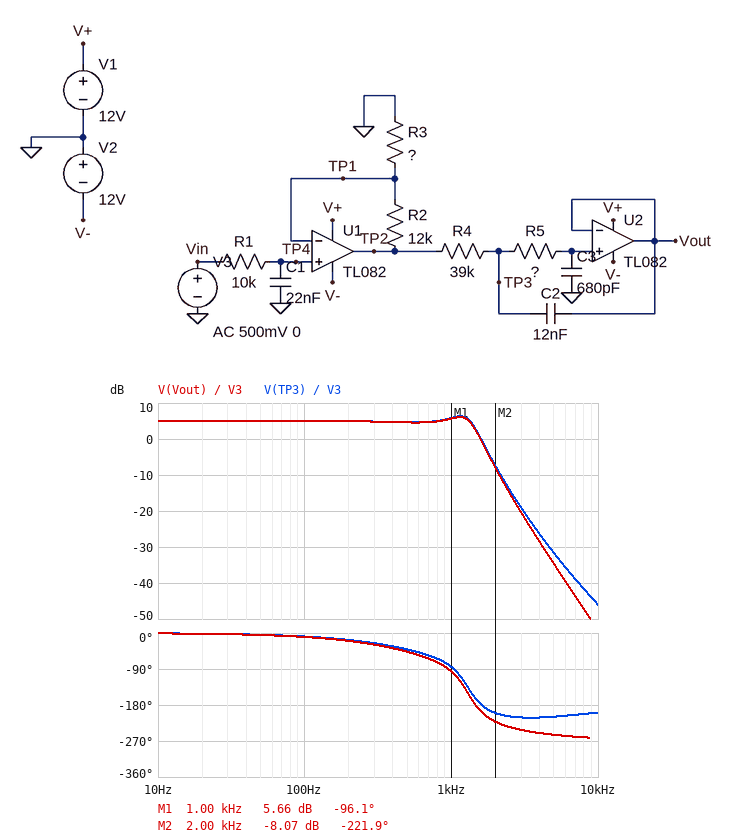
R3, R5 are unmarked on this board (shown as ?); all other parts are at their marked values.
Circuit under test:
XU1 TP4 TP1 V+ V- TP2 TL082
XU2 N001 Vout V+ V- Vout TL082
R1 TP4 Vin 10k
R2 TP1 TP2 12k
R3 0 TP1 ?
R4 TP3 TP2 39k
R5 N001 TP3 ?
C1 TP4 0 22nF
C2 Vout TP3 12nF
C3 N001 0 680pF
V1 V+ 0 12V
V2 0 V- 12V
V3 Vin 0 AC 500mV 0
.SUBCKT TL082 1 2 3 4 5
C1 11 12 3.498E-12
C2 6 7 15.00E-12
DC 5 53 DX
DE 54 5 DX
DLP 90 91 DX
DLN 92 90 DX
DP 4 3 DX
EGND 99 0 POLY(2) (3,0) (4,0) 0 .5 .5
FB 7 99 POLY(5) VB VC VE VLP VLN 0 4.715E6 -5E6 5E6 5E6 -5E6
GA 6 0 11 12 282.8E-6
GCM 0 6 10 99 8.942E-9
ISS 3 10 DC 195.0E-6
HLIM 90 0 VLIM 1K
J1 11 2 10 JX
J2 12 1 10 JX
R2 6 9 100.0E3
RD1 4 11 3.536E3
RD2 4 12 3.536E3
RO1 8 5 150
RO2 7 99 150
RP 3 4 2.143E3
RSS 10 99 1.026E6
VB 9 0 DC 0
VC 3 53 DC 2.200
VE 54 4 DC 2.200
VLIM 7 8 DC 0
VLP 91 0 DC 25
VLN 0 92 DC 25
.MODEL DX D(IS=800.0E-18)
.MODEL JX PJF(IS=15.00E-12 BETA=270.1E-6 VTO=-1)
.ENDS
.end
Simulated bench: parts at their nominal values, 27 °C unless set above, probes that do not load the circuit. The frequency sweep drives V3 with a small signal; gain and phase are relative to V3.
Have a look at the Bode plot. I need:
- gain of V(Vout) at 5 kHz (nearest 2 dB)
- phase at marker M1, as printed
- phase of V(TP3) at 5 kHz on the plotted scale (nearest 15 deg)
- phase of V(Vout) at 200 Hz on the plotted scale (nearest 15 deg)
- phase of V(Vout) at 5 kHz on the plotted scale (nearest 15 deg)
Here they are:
-34 dB
-96.1 deg
-210 deg
-15 deg
-255 deg
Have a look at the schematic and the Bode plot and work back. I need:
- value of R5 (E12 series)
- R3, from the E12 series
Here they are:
47 kΩ
15 kΩ
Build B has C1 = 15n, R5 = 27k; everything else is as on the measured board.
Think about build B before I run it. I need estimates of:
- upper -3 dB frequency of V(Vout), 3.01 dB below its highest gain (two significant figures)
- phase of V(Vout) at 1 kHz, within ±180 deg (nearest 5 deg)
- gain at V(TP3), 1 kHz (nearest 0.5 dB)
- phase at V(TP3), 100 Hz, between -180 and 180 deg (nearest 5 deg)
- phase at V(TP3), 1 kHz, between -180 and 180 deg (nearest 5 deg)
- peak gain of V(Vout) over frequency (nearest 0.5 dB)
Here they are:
1.9 kHz
-65 deg
5.5 dB
-5 deg
-60 deg
6.5 dB
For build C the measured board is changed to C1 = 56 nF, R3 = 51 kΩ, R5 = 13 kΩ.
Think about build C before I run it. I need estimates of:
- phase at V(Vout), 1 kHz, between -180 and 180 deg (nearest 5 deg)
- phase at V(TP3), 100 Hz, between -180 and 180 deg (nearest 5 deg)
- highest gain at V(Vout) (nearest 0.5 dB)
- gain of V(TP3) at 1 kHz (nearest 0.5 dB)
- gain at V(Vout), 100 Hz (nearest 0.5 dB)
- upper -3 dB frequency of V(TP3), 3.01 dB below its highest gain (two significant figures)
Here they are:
-90 deg
-20 deg
2.0 dB
-8.0 dB
1.5 dB
290 Hz
